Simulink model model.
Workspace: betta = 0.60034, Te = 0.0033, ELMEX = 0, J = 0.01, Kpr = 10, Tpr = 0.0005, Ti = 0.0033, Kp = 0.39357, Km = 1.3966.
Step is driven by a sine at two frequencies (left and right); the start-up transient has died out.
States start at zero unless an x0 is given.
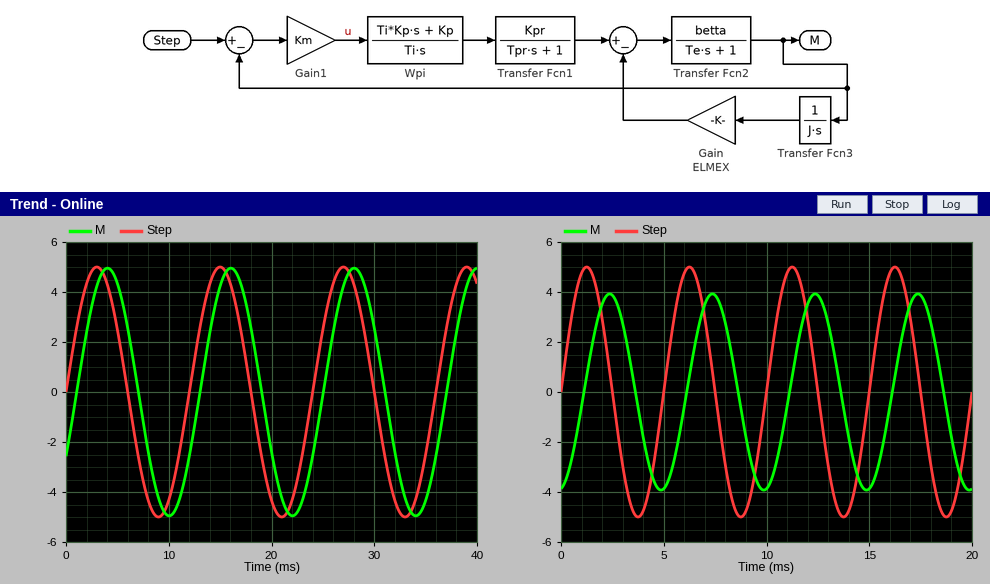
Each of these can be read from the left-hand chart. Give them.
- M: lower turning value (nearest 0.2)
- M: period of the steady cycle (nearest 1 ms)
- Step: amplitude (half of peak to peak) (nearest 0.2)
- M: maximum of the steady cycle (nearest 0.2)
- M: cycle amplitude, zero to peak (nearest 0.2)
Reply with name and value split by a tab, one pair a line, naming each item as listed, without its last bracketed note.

M: lower turning value	-5.0
M: period of the steady cycle	12 ms
Step: amplitude (half of peak to peak)	5.0
M: maximum of the steady cycle	5.0
M: cycle amplitude, zero to peak	5.0
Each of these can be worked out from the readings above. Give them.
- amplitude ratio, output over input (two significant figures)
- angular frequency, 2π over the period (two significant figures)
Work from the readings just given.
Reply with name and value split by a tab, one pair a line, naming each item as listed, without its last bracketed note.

amplitude ratio, output over input	1.0
angular frequency, 2π over the period	0.52 rad/ms
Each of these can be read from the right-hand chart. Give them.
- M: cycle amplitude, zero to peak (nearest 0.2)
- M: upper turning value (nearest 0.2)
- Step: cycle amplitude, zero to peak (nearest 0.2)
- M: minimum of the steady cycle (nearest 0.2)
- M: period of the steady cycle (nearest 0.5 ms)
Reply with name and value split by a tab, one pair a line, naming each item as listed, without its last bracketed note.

M: cycle amplitude, zero to peak	4.0
M: upper turning value	4.0
Step: cycle amplitude, zero to peak	5.0
M: minimum of the steady cycle	-4.0
M: period of the steady cycle	5.0 ms
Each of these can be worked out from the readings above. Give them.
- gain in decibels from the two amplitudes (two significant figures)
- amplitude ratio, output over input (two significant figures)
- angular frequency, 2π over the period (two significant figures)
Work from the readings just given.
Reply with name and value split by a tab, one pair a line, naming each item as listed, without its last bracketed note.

gain in decibels from the two amplitudes	-1.9 dB
amplitude ratio, output over input	0.80
angular frequency, 2π over the period	1.3 rad/ms
